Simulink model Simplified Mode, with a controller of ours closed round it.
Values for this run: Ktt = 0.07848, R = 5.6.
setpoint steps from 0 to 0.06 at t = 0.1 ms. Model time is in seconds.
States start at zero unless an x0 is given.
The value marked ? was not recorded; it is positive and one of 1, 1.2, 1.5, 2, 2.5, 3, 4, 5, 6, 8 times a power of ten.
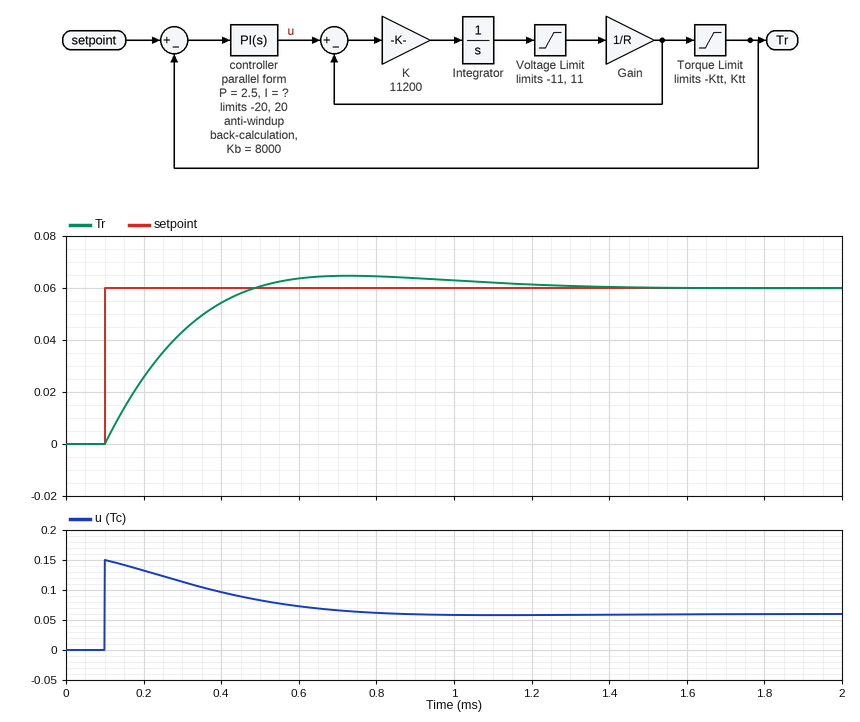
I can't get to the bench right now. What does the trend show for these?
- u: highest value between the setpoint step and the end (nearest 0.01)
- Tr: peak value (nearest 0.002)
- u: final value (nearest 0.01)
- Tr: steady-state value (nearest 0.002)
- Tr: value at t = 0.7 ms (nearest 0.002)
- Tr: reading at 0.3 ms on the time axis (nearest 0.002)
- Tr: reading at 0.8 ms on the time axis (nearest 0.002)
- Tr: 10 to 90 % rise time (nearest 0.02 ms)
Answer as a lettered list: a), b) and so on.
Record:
a) 0.15
b) 0.064
c) 0.06
d) 0.060
e) 0.064
f) 0.044
g) 0.064
h) 0.28 ms
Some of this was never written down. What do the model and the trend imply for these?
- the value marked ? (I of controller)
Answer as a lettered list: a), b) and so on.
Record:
a) 10000
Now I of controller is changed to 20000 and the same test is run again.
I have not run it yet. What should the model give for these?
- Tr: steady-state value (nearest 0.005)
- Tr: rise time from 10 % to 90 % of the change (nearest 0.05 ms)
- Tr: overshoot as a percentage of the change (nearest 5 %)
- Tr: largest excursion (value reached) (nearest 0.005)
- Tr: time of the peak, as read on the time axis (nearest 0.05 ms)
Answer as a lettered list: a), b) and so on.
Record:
a) 0.060
b) 0.20 ms
c) 20 %
d) 0.070
e) 0.55 ms
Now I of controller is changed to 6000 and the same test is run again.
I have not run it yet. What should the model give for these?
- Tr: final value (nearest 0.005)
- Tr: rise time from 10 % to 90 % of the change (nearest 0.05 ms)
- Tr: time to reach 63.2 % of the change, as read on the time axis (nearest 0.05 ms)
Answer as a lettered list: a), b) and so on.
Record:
a) 0.060
b) 0.40 ms
c) 0.30 ms
